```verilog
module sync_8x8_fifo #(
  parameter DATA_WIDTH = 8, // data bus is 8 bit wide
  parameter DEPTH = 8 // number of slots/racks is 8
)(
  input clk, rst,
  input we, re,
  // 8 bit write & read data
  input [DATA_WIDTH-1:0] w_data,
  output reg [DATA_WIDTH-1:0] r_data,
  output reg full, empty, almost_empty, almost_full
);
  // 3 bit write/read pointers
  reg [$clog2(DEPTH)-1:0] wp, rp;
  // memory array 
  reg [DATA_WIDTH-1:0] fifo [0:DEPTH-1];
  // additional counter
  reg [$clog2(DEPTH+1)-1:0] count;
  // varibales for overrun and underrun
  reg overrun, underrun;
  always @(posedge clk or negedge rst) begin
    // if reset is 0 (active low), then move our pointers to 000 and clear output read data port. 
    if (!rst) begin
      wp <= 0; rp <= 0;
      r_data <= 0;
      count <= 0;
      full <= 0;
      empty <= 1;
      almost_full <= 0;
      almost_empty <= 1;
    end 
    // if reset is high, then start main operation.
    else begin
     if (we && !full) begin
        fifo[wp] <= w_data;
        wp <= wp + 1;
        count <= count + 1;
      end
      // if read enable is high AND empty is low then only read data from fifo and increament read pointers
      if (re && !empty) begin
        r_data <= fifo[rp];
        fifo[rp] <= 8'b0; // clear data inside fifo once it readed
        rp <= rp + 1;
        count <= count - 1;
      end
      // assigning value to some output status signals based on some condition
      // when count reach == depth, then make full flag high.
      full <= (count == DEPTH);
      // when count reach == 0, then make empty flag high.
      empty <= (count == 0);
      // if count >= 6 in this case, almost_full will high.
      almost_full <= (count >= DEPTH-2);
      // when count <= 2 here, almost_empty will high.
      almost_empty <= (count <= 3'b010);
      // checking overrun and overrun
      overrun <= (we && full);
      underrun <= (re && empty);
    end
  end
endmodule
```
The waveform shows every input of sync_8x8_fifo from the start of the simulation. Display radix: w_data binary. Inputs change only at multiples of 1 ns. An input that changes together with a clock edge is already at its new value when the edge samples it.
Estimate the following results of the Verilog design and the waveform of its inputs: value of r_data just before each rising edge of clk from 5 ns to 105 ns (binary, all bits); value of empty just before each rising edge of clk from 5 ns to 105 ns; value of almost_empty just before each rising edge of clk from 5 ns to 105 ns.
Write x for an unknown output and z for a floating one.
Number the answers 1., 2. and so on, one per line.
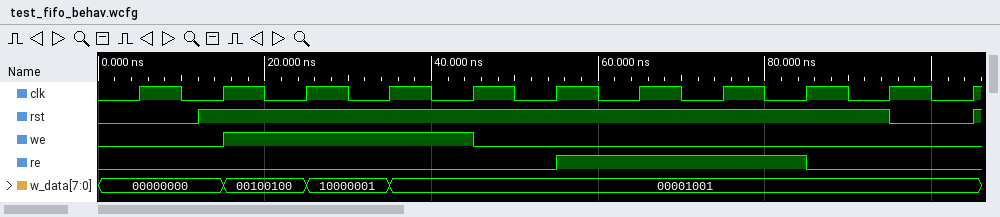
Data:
1. 00000000, 00000000, 00000000, 00000000, 00000000, 00000000, 00100100, 10000001, 00001001, 00001001, 00000000
2. 1 1 1 0 0 0 0 0 0 1 1
3. 1 1 1 1 1 0 0 1 1 1 1
